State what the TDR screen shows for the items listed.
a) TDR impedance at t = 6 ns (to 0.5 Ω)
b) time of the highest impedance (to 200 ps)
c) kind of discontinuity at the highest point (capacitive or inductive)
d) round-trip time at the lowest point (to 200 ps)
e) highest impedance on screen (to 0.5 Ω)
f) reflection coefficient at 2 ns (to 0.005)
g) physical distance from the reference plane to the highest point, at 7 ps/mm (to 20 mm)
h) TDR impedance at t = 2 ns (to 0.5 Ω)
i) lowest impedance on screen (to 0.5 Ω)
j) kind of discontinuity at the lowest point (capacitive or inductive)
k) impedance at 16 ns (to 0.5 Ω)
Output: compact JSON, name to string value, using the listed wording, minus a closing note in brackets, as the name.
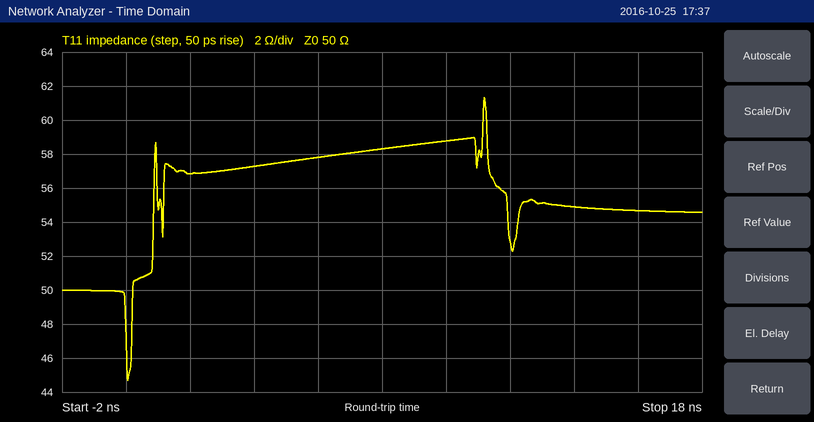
{"TDR impedance at t = 6 ns": "58.0 Ω", "time of the highest impedance": "11.2 ns", "kind of discontinuity at the highest point": "inductive", "round-trip time at the lowest point": "0.0 ns", "highest impedance on screen": "61.5 Ω", "reflection coefficient at 2 ns": "+0.065", "physical distance from the reference plane to the highest point, at 7 ps/mm": "800 mm", "TDR impedance at t = 2 ns": "57.0 Ω", "lowest impedance on screen": "44.5 Ω", "kind of discontinuity at the lowest point": "capacitive", "impedance at 16 ns": "54.5 Ω"}
